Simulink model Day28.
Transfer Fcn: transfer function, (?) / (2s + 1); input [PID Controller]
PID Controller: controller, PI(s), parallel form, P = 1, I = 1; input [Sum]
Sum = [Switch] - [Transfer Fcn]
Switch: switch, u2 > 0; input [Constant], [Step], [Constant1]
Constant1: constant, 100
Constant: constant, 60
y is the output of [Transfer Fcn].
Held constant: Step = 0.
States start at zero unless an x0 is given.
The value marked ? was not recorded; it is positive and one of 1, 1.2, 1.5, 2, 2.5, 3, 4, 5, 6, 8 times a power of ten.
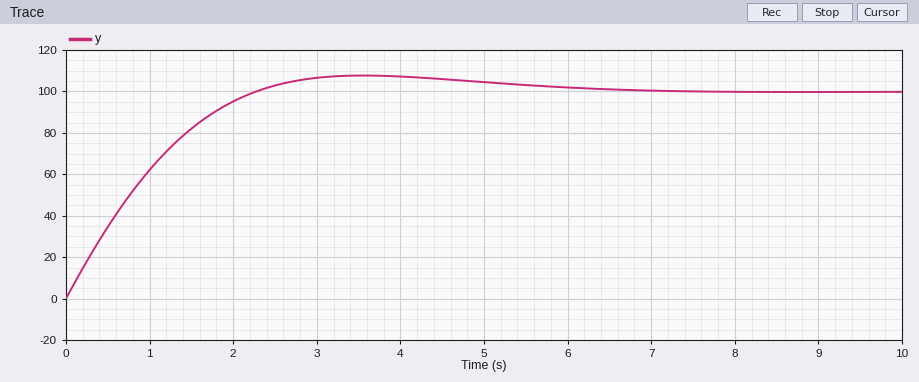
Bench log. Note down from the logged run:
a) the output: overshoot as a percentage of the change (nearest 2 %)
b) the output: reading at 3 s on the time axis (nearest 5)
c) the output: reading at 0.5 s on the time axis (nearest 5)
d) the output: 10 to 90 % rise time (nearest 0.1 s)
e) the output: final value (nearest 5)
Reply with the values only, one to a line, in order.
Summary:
8 %
105
35
1.6 s
100
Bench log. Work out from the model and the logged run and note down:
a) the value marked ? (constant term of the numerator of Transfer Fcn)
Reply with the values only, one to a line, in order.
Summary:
1.5
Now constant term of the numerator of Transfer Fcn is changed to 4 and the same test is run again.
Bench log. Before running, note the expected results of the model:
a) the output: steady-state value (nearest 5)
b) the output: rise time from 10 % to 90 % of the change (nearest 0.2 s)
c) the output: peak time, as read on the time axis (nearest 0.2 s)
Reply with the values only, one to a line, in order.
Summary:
100
0.8 s
1.8 s
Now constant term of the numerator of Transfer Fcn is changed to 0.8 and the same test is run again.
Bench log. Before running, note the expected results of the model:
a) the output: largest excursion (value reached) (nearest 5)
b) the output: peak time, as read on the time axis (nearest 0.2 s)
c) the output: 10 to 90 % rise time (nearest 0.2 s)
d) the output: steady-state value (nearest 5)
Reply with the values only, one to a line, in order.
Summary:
105
5.6 s
2.6 s
100
